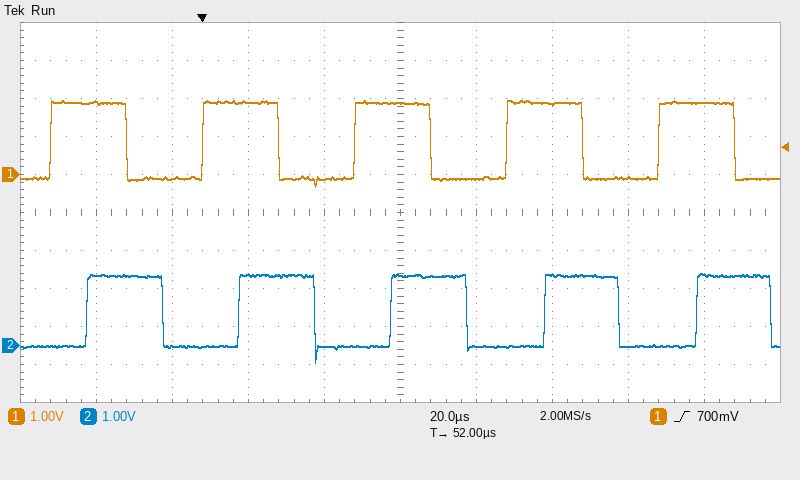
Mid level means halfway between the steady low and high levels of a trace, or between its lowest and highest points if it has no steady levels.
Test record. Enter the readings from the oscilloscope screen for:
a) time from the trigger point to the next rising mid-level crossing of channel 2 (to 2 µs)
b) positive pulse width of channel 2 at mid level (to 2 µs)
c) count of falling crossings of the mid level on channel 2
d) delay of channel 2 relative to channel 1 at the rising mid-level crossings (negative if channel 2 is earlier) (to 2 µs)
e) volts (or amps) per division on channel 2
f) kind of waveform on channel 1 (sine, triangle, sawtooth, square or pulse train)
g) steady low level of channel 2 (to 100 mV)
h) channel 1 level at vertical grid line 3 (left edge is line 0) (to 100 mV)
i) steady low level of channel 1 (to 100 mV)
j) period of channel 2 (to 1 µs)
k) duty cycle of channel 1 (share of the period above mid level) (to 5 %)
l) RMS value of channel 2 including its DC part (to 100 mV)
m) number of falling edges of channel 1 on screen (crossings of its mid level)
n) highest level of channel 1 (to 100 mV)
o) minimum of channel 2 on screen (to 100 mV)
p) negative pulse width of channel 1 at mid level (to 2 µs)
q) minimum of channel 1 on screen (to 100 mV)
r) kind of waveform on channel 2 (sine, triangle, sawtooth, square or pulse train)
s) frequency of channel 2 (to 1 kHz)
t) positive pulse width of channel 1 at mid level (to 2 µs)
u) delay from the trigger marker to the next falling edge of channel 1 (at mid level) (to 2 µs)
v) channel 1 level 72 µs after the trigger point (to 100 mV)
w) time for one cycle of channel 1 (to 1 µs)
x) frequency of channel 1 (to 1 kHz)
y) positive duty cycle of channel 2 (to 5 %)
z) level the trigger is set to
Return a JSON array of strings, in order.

["10 µs", "20 µs", "5", "+10 µs", "1 V", "square", "0.0 V", "1.9 V", "-100 mV", "40 µs", "50 %", "1.3 V", "5", "1.9 V", "-400 mV", "20 µs", "-300 mV", "square", "25 kHz", "20 µs", "20 µs", "-100 mV", "40 µs", "25 kHz", "50 %", "700 mV"]
